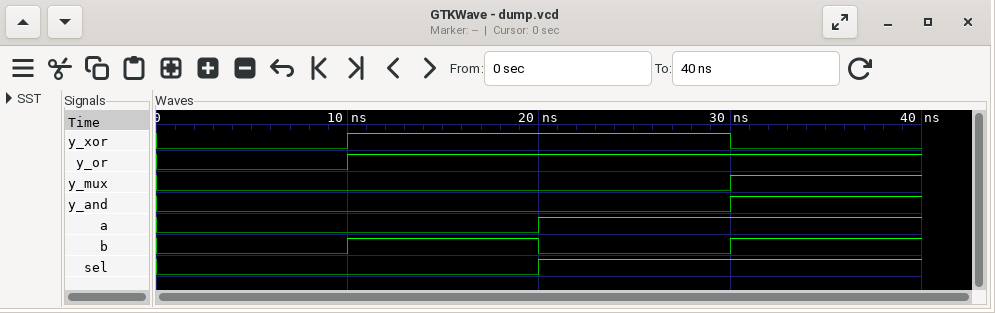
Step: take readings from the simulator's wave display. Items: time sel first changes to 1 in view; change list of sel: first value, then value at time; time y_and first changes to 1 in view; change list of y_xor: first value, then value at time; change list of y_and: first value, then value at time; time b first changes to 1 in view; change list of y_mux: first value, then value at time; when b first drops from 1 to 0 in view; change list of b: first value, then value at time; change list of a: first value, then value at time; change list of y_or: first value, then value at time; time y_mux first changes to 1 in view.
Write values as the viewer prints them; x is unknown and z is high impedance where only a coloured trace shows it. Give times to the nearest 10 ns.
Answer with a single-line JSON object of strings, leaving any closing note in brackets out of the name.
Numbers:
{"time sel first changes to 1 in view": "20 ns", "change list of sel: first value, then value at time": "0, 1 at 20 ns", "time y_and first changes to 1 in view": "30 ns", "change list of y_xor: first value, then value at time": "0, 1 at 10 ns, 0 at 30 ns", "change list of y_and: first value, then value at time": "0, 1 at 30 ns", "time b first changes to 1 in view": "10 ns", "change list of y_mux: first value, then value at time": "0, 1 at 30 ns", "when b first drops from 1 to 0 in view": "20 ns", "change list of b: first value, then value at time": "0, 1 at 10 ns, 0 at 20 ns, 1 at 30 ns", "change list of a: first value, then value at time": "0, 1 at 20 ns", "change list of y_or: first value, then value at time": "0, 1 at 10 ns", "time y_mux first changes to 1 in view": "30 ns"}
